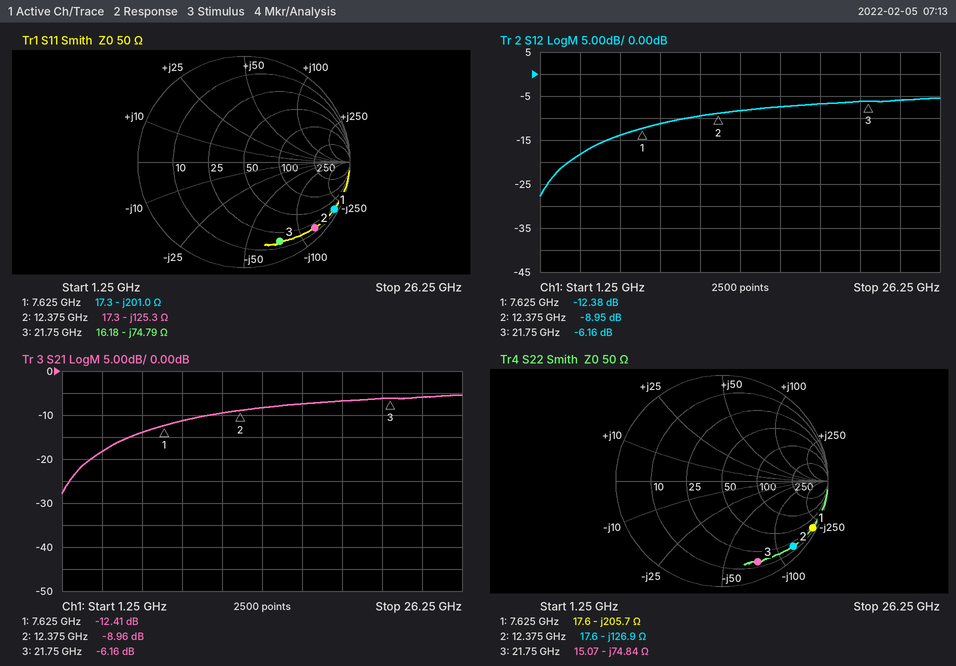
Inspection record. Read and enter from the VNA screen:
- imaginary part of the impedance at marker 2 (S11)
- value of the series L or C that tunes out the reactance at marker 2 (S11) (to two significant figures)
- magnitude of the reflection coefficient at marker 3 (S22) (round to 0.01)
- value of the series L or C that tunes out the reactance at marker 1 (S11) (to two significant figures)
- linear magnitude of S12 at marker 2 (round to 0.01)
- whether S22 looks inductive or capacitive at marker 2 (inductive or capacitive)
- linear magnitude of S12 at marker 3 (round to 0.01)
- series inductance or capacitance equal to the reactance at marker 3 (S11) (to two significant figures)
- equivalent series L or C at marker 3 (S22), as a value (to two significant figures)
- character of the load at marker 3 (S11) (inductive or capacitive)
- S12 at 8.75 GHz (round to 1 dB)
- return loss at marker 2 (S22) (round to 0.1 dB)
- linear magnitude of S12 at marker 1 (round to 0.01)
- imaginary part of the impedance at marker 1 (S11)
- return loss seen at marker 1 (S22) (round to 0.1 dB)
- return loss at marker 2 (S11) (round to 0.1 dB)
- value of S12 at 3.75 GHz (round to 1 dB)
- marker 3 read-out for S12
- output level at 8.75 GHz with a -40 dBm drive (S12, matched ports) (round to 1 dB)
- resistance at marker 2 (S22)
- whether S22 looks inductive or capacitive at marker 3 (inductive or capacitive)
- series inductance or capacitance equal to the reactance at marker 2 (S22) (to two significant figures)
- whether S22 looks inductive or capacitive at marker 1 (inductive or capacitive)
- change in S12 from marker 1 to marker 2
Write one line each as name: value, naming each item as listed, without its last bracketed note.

imaginary part of the impedance at marker 2: -125.3 Ω
value of the series L or C that tunes out the reactance at marker 2 (S11): 1.6 nH
magnitude of the reflection coefficient at marker 3 (S22): 0.83
value of the series L or C that tunes out the reactance at marker 1 (S11): 4.2 nH
linear magnitude of S12 at marker 2: 0.36
whether S22 looks inductive or capacitive at marker 2: capacitive
linear magnitude of S12 at marker 3: 0.49
series inductance or capacitance equal to the reactance at marker 3 (S11): 98 fF
equivalent series L or C at marker 3 (S22), as a value: 98 fF
character of the load at marker 3 (S11): capacitive
S12 at 8.75 GHz: -11 dB
return loss at marker 2 (S22): 0.8 dB
linear magnitude of S12 at marker 1: 0.24
imaginary part of the impedance at marker 1: -201.0 Ω
return loss seen at marker 1 (S22): 0.3 dB
return loss at marker 2 (S11): 0.8 dB
value of S12 at 3.75 GHz: -18 dB
marker 3 read-out for S12: -6.16 dB
output level at 8.75 GHz with a -40 dBm drive (S12, matched ports): -51 dBm
resistance at marker 2: 17.6 Ω
whether S22 looks inductive or capacitive at marker 3: capacitive
series inductance or capacitance equal to the reactance at marker 2 (S22): 100 fF
whether S22 looks inductive or capacitive at marker 1: capacitive
change in S12 from marker 1 to marker 2: 3.43 dB
